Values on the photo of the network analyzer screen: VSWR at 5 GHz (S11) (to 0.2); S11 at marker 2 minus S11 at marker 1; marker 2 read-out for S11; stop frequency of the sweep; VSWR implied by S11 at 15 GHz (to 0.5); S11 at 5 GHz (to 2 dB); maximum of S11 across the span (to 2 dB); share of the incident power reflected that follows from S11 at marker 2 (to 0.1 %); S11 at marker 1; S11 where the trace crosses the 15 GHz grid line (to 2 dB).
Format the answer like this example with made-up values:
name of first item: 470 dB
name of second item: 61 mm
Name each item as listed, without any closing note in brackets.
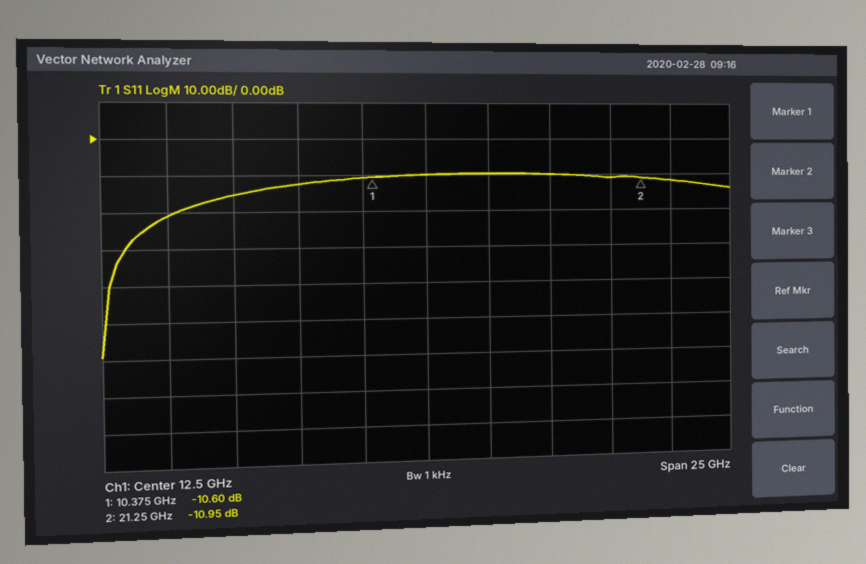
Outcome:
VSWR at 5 GHz (S11): 1.4
S11 at marker 2 minus S11 at marker 1: -0.35 dB
marker 2 read-out for S11: -10.95 dB
stop frequency of the sweep: 25 GHz
VSWR implied by S11 at 15 GHz: 2.0
S11 at 5 GHz: -16 dB
maximum of S11 across the span: -10 dB
share of the incident power reflected that follows from S11 at marker 2: 8.0 %
S11 at marker 1: -10.60 dB
S11 where the trace crosses the 15 GHz grid line: -10 dB
